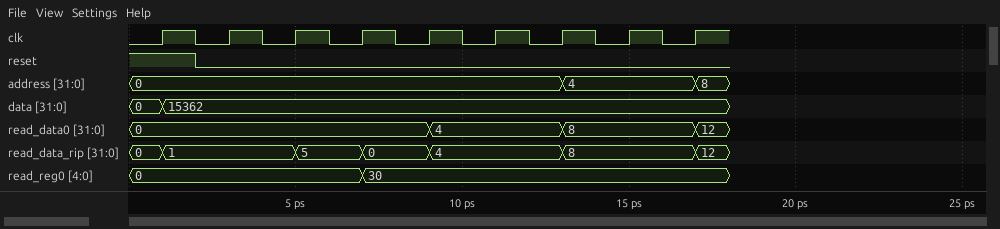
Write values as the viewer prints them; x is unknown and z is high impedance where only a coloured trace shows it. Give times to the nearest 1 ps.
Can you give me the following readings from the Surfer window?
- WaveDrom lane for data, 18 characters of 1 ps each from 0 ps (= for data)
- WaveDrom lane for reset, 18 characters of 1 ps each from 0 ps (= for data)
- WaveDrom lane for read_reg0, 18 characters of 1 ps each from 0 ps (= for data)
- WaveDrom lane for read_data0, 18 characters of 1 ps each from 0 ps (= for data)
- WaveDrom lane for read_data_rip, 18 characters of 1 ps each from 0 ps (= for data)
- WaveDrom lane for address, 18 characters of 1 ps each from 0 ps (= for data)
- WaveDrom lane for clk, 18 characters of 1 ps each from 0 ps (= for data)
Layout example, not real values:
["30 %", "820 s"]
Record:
["{name: 'data', wave: '==................', data: '0 15362'}", "{name: 'reset', wave: '1.0...............'}", "{name: 'read_reg0', wave: '=......=..........', data: '0 30'}", "{name: 'read_data0', wave: '=........=...=...=', data: '0 4 8 12'}", "{name: 'read_data_rip', wave: '==...=.=.=...=...=', data: '0 1 5 0 4 8 12'}", "{name: 'address', wave: '=............=...=', data: '0 4 8'}", "{name: 'clk', wave: '010101010101010101'}"]
